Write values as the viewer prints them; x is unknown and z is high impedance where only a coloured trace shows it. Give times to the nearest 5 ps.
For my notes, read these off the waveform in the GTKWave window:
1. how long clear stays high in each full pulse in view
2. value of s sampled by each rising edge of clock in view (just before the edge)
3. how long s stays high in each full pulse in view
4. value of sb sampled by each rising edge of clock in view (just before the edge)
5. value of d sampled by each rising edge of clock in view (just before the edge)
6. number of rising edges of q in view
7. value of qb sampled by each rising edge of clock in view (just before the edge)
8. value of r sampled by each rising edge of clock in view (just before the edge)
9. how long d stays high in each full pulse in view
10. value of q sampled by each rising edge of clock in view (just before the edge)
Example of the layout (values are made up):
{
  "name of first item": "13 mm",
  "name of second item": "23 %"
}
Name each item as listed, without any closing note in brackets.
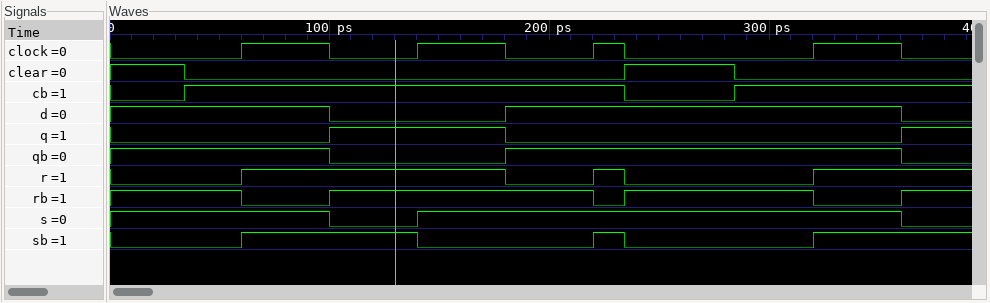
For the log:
{
  "how long clear stays high in each full pulse in view": "50 ps",
  "value of s sampled by each rising edge of clock in view": "1 0 1 1",
  "how long s stays high in each full pulse in view": "220 ps",
  "value of sb sampled by each rising edge of clock in view": "0 1 0 0",
  "value of d sampled by each rising edge of clock in view": "1 0 1 1",
  "number of rising edges of q in view": "2",
  "value of qb sampled by each rising edge of clock in view": "1 0 1 1",
  "value of r sampled by each rising edge of clock in view": "0 1 0 0",
  "how long d stays high in each full pulse in view": "180 ps",
  "value of q sampled by each rising edge of clock in view": "0 1 0 0"
}
